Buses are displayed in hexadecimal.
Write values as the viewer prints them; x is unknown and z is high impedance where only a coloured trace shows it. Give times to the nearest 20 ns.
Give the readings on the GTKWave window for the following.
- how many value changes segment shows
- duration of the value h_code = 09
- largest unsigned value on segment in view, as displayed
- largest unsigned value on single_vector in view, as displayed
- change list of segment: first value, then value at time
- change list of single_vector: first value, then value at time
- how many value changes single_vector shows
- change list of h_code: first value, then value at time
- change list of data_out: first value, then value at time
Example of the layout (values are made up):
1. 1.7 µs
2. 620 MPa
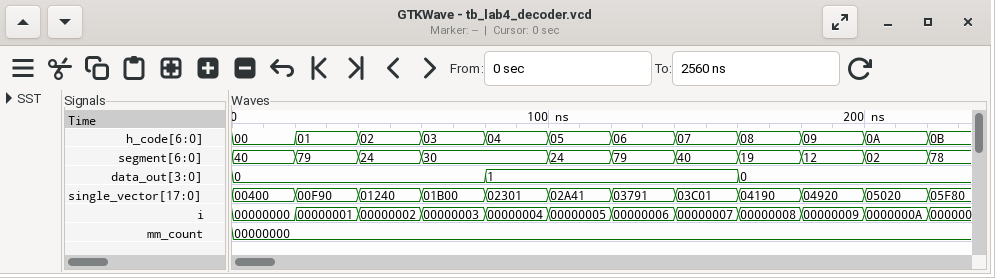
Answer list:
1. 10
2. 20 ns
3. 79
4. 05F80
5. 40, 79 at 20 ns, 24 at 40 ns, 30 at 60 ns, 24 at 100 ns, 79 at 120 ns, 40 at 140 ns, 19 at 160 ns, 12 at 180 ns, 02 at 200 ns, 78 at 220 ns
6. 00400, 00F90 at 20 ns, 01240 at 40 ns, 01B00 at 60 ns, 02301 at 80 ns, 02A41 at 100 ns, 03791 at 120 ns, 03C01 at 140 ns, 04190 at 160 ns, 04920 at 180 ns, 05020 at 200 ns, 05F80 at 220 ns
7. 11
8. 00, 01 at 20 ns, 02 at 40 ns, 03 at 60 ns, 04 at 80 ns, 05 at 100 ns, 06 at 120 ns, 07 at 140 ns, 08 at 160 ns, 09 at 180 ns, 0A at 200 ns, 0B at 220 ns
9. 0, 1 at 80 ns, 0 at 160 ns
